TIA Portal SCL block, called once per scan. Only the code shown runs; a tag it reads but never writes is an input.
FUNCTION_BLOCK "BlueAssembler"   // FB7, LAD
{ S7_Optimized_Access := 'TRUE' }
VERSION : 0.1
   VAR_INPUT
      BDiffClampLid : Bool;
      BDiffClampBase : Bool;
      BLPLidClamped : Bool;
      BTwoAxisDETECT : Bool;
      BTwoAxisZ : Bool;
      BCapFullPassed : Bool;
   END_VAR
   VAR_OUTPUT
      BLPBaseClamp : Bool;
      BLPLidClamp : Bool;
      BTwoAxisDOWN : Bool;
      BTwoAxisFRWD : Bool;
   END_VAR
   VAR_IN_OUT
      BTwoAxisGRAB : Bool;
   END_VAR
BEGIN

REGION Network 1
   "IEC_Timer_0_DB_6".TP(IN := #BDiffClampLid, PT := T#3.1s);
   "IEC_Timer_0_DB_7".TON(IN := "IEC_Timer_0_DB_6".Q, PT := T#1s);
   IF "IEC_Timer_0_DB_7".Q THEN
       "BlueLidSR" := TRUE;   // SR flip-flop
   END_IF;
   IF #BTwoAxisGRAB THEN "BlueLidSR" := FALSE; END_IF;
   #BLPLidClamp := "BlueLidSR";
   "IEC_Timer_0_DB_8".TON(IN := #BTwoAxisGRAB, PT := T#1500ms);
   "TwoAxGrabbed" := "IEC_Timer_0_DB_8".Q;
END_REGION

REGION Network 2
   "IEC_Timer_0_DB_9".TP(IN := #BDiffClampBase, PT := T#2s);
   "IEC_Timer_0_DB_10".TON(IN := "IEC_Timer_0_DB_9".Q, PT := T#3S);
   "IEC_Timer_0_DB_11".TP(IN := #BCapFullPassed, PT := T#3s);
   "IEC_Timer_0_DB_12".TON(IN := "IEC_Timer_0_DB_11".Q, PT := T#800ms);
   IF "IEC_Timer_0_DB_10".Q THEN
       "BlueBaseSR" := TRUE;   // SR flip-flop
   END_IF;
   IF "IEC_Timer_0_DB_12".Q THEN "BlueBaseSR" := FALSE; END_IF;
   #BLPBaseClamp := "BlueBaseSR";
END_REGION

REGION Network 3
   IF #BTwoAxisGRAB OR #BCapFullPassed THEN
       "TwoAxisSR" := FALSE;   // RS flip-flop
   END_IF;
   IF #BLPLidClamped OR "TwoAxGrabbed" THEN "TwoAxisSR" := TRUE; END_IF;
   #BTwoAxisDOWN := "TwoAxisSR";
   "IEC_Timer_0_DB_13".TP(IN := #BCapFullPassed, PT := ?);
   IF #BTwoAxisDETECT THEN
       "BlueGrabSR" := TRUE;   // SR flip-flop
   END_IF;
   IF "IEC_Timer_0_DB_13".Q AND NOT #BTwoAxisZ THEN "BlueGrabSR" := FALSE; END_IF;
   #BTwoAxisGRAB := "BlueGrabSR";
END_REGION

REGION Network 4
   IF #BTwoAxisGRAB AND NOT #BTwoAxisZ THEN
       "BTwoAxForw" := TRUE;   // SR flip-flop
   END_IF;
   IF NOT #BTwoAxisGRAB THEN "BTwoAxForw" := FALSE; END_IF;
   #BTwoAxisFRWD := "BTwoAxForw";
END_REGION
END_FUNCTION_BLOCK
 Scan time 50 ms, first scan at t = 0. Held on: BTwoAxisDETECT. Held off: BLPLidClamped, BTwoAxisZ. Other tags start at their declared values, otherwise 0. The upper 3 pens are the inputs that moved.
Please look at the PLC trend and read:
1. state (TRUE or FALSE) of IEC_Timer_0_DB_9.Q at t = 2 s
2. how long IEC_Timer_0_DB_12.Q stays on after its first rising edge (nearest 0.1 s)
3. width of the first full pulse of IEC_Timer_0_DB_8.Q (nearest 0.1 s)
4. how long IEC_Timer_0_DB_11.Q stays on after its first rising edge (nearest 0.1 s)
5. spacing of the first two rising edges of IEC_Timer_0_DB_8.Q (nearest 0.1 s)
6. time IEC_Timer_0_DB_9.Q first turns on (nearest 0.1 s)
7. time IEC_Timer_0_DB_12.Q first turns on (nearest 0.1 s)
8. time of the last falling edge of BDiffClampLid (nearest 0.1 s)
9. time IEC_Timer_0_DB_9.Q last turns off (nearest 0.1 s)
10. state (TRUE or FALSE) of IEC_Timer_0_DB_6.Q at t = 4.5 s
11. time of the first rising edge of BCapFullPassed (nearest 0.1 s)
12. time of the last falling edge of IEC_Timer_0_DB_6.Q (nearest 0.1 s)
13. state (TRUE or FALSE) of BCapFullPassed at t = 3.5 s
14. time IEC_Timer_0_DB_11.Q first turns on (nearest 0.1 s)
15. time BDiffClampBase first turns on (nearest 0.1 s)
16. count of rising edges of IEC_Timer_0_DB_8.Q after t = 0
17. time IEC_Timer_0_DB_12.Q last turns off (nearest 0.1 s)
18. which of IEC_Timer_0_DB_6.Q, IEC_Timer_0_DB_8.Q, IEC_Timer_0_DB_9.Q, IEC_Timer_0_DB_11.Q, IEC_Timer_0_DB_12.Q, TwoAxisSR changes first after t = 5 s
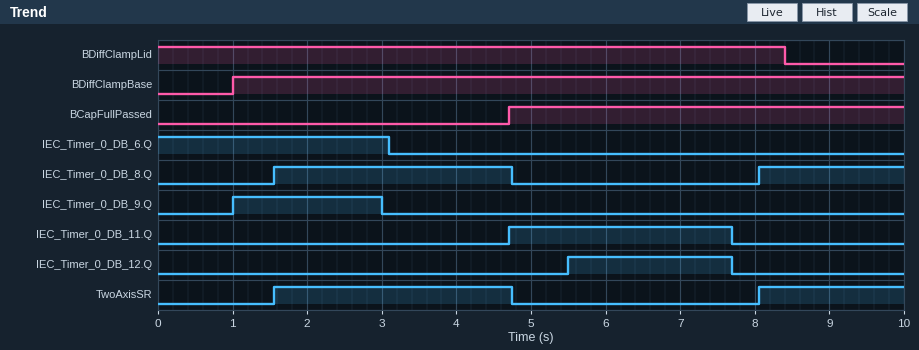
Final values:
TRUE
2.2 s
3.2 s
3.0 s
6.5 s
1.0 s
5.5 s
8.4 s
3.0 s
FALSE
4.7 s
3.1 s
FALSE
4.7 s
1.0 s
2
7.7 s
IEC_Timer_0_DB_12.Q
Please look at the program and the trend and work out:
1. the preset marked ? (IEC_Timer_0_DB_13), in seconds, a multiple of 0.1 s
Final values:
1.8 s
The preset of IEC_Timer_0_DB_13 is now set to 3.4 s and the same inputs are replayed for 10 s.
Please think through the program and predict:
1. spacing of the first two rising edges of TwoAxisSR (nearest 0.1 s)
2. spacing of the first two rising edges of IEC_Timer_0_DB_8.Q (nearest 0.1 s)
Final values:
8.1 s
8.1 s
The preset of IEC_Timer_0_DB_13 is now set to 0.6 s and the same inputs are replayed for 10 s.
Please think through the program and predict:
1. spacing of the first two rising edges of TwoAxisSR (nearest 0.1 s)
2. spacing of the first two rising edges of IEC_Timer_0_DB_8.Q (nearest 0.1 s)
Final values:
5.3 s
5.3 s
